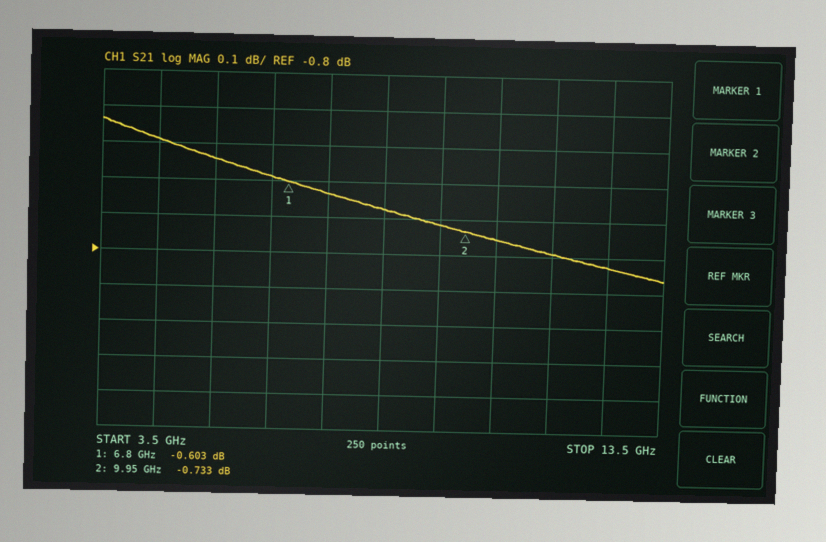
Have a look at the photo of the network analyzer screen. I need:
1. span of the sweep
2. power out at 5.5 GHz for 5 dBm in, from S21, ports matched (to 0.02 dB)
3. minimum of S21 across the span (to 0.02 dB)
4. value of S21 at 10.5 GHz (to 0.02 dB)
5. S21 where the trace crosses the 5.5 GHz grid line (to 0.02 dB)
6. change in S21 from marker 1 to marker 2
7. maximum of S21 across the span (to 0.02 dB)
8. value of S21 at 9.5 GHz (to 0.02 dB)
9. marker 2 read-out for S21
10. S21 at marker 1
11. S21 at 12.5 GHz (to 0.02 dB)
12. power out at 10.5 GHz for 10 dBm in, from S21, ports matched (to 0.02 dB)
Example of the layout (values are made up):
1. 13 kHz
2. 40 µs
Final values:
1. 10 GHz
2. 4.46 dBm
3. -0.86 dB
4. -0.76 dB
5. -0.54 dB
6. -0.130 dB
7. -0.44 dB
8. -0.72 dB
9. -0.733 dB
10. -0.603 dB
11. -0.82 dB
12. 9.24 dBm
